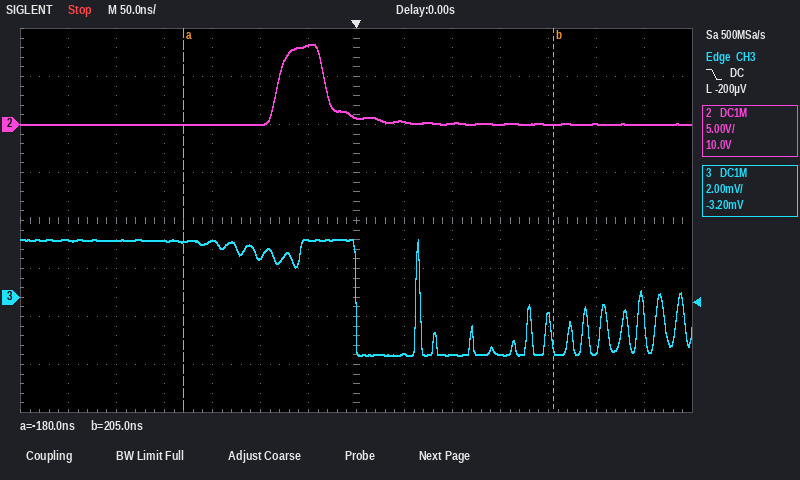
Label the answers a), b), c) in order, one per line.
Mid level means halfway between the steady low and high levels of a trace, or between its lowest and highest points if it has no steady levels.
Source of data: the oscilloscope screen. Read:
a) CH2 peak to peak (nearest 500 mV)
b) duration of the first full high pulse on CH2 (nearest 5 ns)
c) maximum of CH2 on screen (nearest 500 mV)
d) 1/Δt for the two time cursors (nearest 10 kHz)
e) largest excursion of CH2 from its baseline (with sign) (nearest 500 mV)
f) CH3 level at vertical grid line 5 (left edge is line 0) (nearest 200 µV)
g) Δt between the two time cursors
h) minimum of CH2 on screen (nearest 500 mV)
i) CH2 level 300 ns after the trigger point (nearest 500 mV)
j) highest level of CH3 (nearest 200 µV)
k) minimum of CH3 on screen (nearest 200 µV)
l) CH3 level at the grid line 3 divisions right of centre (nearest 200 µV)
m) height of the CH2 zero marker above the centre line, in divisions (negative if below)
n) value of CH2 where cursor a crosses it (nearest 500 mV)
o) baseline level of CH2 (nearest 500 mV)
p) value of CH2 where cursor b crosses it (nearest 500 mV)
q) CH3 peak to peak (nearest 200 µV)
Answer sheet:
a) 8.5 V
b) 50 ns
c) 8.5 V
d) 2.60 MHz
e) +8.5 V
f) 1.6 mV
g) 385 ns
h) 0.0 V
i) 0.0 V
j) 2.4 mV
k) -2.4 mV
l) -2.4 mV
m) +2.0 div
n) 0.0 V
o) 0.0 V
p) 0.0 V
q) 4.8 mV
